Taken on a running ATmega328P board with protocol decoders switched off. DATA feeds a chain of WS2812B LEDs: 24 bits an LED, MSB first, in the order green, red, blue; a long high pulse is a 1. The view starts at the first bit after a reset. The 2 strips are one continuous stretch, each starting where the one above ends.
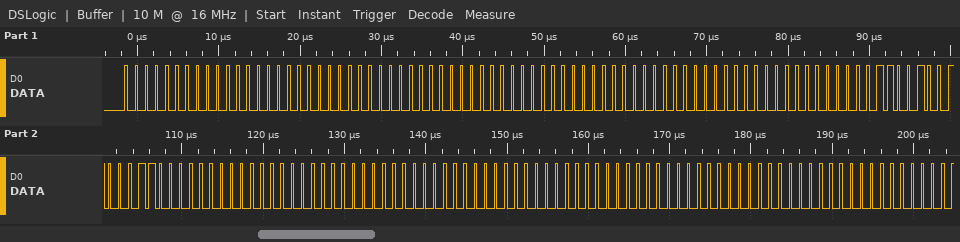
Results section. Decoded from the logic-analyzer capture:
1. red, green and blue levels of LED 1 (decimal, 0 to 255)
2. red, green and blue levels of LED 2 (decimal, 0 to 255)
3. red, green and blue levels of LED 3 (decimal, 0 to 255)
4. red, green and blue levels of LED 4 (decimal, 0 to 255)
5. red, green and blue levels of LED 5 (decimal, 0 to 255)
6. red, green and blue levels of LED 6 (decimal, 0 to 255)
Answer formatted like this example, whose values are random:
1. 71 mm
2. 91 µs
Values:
1. 0, 0, 0
2. 0, 0, 0
3. 0, 0, 0
4. 70, 50, 0
5. 0, 0, 0
6. 0, 0, 0
